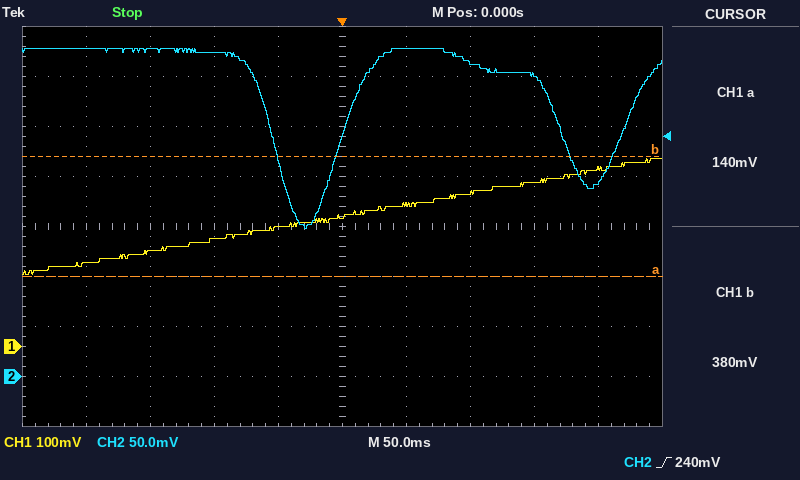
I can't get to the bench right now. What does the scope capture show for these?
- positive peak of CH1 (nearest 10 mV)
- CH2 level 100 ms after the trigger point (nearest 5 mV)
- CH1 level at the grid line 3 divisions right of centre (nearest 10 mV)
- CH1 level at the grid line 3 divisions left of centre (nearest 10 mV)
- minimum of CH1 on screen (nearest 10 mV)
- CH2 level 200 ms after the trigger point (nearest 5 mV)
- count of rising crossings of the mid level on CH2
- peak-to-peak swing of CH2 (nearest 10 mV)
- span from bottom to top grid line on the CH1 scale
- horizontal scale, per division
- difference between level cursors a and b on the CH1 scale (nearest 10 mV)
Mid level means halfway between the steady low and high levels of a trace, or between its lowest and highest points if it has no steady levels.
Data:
380 mV
315 mV
330 mV
190 mV
140 mV
195 mV
2
180 mV
800 mV
50 ms
240 mV
